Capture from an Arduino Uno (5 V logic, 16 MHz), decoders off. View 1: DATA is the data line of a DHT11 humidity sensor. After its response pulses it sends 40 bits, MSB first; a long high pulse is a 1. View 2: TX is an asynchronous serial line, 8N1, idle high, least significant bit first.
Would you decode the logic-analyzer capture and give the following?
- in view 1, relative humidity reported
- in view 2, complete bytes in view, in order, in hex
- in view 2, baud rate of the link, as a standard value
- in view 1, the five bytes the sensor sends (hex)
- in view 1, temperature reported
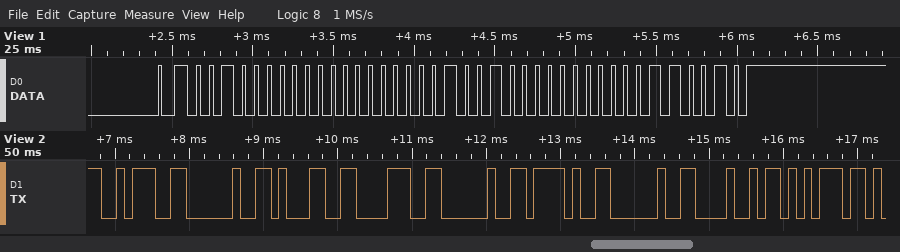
32 %
3A 20 31 38 20 2F 20 48 75
9600 baud
20 00 12 00 32
18.0 °C
